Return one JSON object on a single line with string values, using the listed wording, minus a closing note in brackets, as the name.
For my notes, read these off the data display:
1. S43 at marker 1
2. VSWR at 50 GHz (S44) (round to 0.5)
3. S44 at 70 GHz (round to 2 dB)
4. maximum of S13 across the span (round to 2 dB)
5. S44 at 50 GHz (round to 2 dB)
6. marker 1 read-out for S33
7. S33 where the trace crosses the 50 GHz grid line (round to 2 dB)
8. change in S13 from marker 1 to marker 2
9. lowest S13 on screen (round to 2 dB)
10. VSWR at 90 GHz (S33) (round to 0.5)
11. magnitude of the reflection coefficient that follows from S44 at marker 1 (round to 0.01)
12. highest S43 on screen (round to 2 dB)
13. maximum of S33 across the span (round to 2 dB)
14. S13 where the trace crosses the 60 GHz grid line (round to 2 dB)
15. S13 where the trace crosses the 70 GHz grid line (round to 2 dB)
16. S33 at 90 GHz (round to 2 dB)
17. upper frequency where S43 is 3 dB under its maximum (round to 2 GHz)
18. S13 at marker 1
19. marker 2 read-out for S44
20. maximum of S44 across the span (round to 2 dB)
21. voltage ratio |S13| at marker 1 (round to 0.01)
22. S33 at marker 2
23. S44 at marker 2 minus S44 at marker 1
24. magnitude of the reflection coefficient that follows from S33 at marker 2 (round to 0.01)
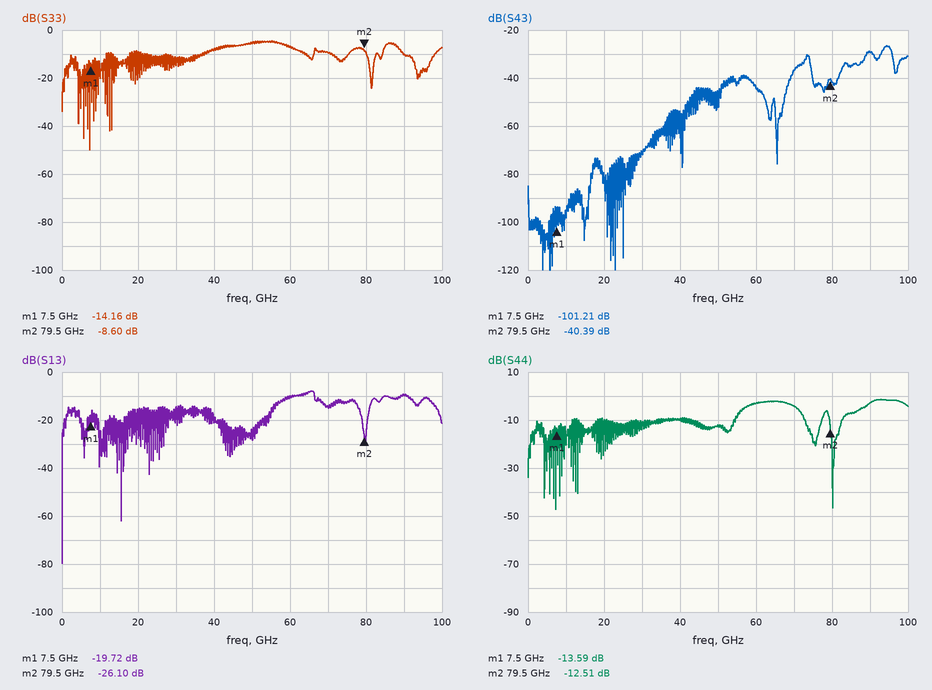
{"S43 at marker 1": "-101.21 dB", "VSWR at 50 GHz (S44)": "1.5", "S44 at 70 GHz": "-4 dB", "maximum of S13 across the span": "-8 dB", "S44 at 50 GHz": "-12 dB", "marker 1 read-out for S33": "-14.16 dB", "S33 where the trace crosses the 50 GHz grid line": "-6 dB", "change in S13 from marker 1 to marker 2": "-6.38 dB", "lowest S13 on screen": "-80 dB", "VSWR at 90 GHz (S33)": "2.0", "magnitude of the reflection coefficient that follows from S44 at marker 1": "0.21", "highest S43 on screen": "-26 dB", "maximum of S33 across the span": "-4 dB", "S13 where the trace crosses the 60 GHz grid line": "-10 dB", "S13 where the trace crosses the 70 GHz grid line": "-14 dB", "S33 at 90 GHz": "-10 dB", "upper frequency where S43 is 3 dB under its maximum": "96 GHz", "S13 at marker 1": "-19.72 dB", "marker 2 read-out for S44": "-12.51 dB", "maximum of S44 across the span": "-2 dB", "voltage ratio |S13| at marker 1": "0.10", "S33 at marker 2": "-8.60 dB", "S44 at marker 2 minus S44 at marker 1": "1.08 dB", "magnitude of the reflection coefficient that follows from S33 at marker 2": "0.37"}
